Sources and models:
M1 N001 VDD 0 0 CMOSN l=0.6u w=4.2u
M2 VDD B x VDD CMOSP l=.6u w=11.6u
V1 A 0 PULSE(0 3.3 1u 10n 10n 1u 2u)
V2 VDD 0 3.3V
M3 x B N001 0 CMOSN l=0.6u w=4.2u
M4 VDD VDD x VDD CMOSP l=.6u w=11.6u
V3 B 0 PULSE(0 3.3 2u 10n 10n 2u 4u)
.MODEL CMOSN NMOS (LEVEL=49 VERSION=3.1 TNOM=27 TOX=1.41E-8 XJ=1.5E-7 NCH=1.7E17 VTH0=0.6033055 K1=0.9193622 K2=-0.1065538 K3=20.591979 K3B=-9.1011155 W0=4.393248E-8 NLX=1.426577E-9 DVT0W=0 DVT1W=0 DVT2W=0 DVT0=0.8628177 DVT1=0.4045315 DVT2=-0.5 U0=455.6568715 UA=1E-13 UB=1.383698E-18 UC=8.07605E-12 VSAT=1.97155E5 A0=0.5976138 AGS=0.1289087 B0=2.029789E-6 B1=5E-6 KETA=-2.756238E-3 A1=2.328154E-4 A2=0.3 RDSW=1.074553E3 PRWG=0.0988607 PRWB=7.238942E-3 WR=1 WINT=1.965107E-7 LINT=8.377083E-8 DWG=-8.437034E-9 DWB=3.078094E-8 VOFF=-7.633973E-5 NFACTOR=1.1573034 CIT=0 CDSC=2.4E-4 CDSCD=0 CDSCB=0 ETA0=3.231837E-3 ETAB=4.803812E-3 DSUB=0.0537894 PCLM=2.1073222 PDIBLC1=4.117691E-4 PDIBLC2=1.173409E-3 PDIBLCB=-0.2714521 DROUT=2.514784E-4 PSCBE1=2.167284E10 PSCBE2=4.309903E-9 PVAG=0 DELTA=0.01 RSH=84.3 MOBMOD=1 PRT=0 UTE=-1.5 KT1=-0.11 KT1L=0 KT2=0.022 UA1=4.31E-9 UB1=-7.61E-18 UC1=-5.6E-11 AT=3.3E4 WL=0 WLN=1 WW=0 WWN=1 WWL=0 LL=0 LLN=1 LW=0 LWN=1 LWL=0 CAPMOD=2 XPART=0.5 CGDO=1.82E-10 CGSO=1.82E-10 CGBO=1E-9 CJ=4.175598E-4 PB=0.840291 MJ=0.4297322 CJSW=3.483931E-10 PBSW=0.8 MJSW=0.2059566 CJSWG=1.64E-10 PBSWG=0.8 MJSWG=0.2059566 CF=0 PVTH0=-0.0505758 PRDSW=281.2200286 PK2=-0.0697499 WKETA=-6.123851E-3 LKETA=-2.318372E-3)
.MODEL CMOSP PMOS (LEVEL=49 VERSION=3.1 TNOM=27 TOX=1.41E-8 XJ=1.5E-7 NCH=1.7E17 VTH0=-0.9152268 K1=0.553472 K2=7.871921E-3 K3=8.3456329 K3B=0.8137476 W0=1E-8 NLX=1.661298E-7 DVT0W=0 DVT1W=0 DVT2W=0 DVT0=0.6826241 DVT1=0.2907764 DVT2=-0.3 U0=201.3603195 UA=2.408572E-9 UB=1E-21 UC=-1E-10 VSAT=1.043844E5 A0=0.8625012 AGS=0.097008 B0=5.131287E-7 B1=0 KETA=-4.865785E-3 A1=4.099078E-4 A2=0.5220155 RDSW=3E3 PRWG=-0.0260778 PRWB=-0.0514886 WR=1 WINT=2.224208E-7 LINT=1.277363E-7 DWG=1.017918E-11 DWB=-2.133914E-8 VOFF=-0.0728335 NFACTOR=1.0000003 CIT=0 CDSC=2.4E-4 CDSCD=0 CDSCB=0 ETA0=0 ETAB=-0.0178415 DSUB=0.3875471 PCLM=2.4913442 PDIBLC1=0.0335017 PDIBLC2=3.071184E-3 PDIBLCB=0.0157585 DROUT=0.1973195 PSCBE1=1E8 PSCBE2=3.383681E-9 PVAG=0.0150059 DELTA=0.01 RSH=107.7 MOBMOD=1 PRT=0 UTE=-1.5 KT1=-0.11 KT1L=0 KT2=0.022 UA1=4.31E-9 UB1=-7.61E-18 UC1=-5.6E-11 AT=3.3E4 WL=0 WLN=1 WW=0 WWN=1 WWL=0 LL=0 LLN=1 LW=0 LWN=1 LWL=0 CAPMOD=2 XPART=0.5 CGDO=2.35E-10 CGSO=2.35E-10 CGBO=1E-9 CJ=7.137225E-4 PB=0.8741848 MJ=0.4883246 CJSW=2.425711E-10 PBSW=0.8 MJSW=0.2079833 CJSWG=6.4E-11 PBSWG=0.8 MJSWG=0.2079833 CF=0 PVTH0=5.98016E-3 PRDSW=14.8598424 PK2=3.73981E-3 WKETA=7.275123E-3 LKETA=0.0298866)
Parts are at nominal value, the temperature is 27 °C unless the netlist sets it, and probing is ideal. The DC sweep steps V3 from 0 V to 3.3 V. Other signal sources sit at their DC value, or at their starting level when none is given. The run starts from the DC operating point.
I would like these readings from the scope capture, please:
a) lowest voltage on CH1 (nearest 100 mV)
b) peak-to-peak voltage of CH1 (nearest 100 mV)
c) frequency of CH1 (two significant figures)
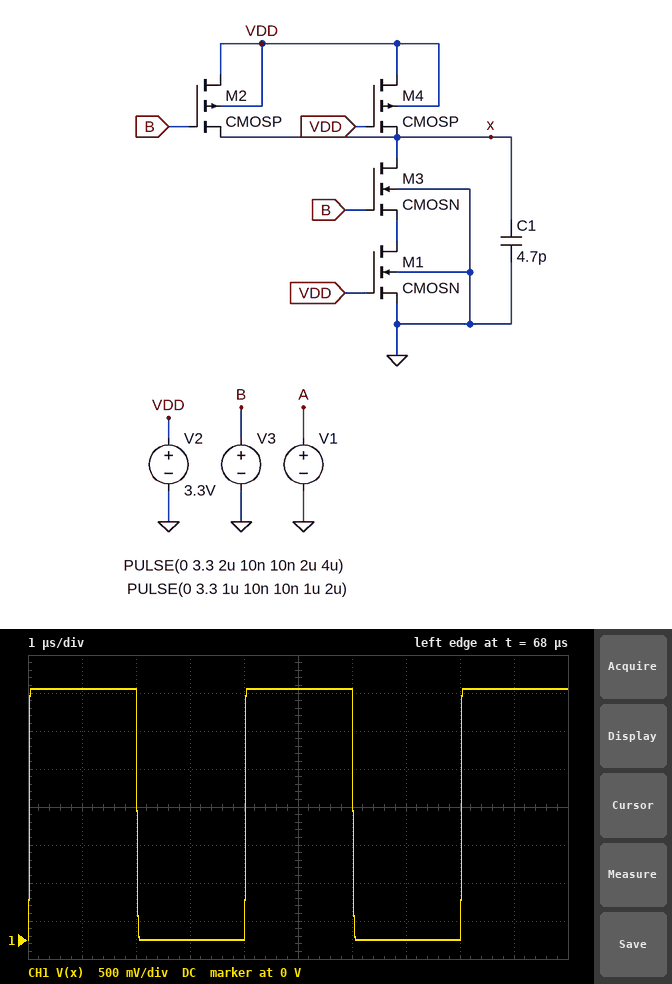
0 V
3.3 V
250 kHz
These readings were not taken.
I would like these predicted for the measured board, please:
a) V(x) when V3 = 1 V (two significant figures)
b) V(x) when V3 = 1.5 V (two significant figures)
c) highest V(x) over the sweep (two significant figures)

3.2 V
3.0 V
3.3 V
